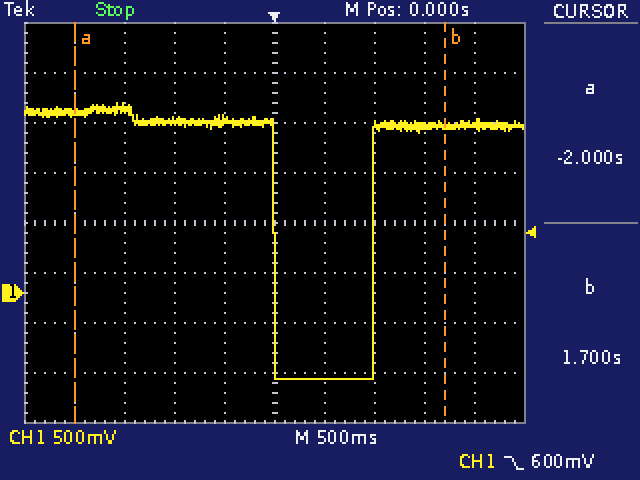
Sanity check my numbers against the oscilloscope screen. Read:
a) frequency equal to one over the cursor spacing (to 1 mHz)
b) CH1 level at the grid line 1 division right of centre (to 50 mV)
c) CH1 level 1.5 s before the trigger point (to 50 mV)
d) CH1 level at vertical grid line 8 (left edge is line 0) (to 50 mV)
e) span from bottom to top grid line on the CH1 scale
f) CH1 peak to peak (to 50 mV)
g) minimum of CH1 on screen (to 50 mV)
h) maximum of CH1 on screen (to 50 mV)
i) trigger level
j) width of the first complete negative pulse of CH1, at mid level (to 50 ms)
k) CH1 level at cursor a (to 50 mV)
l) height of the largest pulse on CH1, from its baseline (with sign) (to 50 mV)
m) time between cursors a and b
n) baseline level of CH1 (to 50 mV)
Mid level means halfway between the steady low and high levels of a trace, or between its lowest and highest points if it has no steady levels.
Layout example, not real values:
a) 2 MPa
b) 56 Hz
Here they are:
a) 270 mHz
b) -850 mV
c) 1.85 V
d) 1.65 V
e) 4 V
f) 2.75 V
g) -850 mV
h) 1.90 V
i) 600 mV
j) 1.00 s
k) 1.80 V
l) -2.55 V
m) 3.70 s
n) 1.70 V
